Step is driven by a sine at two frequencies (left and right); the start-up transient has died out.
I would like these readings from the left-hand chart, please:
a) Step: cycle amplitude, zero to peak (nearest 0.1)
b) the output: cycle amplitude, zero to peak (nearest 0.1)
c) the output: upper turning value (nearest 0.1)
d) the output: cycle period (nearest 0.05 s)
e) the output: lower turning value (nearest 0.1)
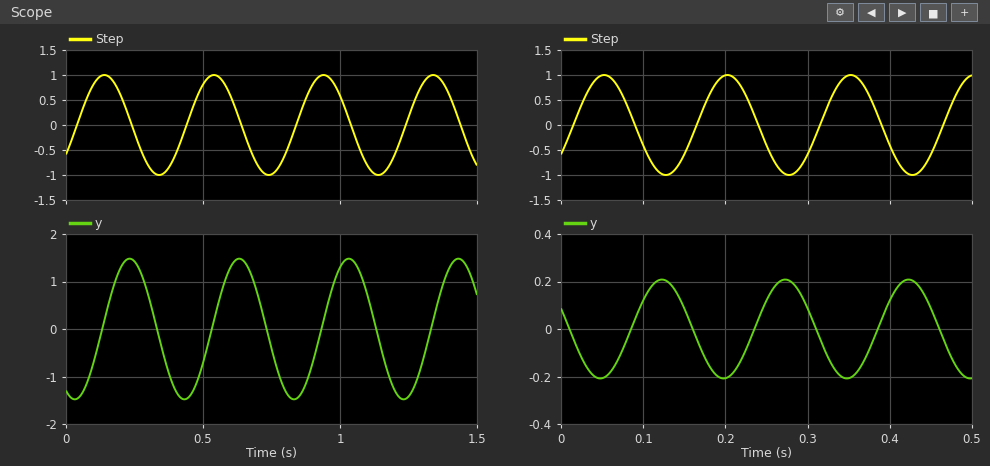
1.0
1.5
1.5
0.40 s
-1.5
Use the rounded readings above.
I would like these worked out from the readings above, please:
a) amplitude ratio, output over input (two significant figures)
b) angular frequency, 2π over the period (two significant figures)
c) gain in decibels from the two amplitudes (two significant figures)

1.5
16 rad/s
3.5 dB
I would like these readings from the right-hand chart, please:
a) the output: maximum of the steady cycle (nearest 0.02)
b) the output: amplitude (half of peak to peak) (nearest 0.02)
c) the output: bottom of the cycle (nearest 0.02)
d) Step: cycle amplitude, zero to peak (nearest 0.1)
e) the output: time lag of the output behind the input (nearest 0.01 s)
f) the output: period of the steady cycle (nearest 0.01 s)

0.20
0.20
-0.20
1.0
0.07 s
0.15 s
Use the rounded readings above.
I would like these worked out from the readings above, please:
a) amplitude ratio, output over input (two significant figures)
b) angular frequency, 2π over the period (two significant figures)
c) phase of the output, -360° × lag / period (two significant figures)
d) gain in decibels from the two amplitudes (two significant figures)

0.20
42 rad/s
-170°
-14 dB
